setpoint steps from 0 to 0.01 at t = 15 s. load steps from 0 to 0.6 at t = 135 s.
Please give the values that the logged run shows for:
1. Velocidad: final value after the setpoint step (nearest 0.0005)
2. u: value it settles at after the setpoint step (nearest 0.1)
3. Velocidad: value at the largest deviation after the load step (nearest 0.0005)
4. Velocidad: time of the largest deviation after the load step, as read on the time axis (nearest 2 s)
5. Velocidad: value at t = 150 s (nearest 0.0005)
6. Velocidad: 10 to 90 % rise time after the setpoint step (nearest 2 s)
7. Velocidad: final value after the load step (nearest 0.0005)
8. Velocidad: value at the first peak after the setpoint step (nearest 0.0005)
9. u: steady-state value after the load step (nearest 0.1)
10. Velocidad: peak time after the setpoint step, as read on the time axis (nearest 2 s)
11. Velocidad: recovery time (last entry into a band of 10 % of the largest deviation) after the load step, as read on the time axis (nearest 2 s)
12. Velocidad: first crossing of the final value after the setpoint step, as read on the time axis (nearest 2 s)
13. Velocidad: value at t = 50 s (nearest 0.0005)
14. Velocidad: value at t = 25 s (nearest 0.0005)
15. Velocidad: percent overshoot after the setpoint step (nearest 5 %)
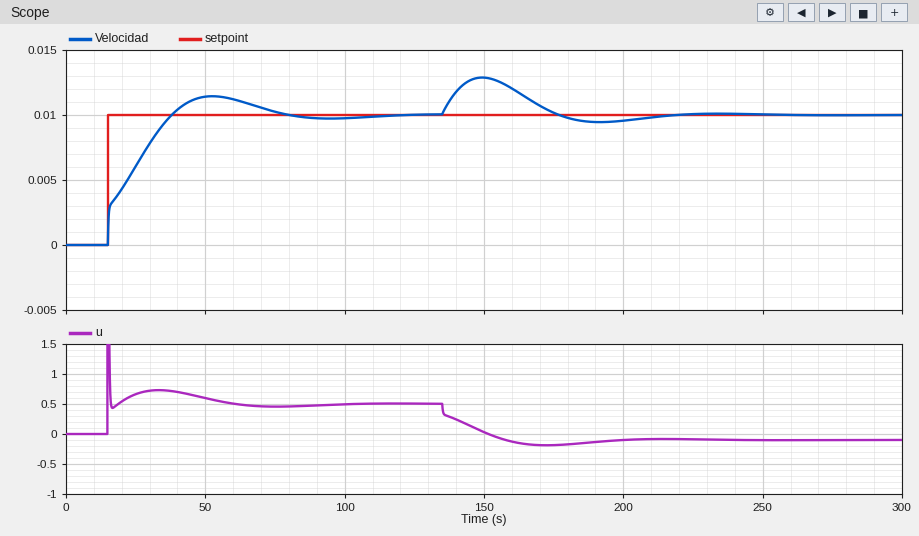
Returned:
0.0100
0.5
0.0130
150 s
0.0130
18 s
0.0100
0.0115
-0.1
52 s
206 s
38 s
0.0115
0.0060
15 %
